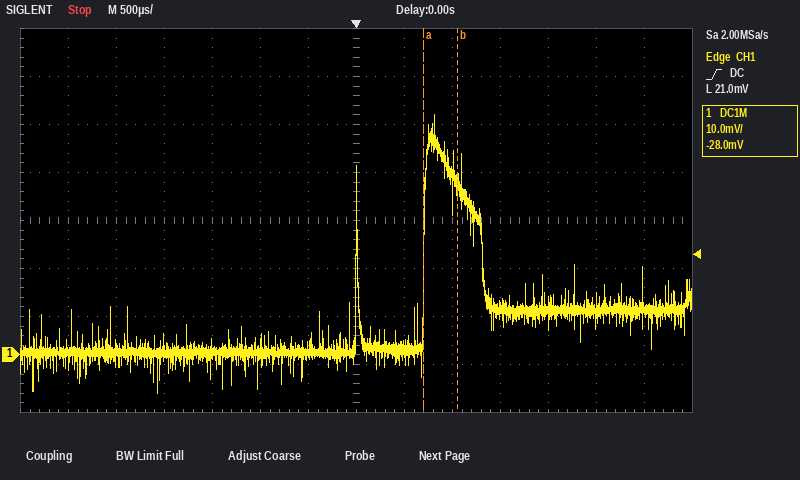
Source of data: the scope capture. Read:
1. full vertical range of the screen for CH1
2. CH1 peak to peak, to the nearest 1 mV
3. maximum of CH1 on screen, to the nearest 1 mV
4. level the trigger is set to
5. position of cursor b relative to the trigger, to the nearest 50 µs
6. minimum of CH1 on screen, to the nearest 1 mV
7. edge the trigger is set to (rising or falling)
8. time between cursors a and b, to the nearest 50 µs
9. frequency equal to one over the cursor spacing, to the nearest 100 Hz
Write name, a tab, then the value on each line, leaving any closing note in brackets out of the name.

full vertical range of the screen for CH1	80 mV
CH1 peak to peak, to the nearest 1 mV	58 mV
maximum of CH1 on screen, to the nearest 1 mV	50 mV
level the trigger is set to	21.0 mV
position of cursor b relative to the trigger, to the nearest 50 µs	+1.05 ms
minimum of CH1 on screen, to the nearest 1 mV	-8 mV
edge the trigger is set to	rising
time between cursors a and b, to the nearest 50 µs	350 µs
frequency equal to one over the cursor spacing, to the nearest 100 Hz	2.9 kHz
